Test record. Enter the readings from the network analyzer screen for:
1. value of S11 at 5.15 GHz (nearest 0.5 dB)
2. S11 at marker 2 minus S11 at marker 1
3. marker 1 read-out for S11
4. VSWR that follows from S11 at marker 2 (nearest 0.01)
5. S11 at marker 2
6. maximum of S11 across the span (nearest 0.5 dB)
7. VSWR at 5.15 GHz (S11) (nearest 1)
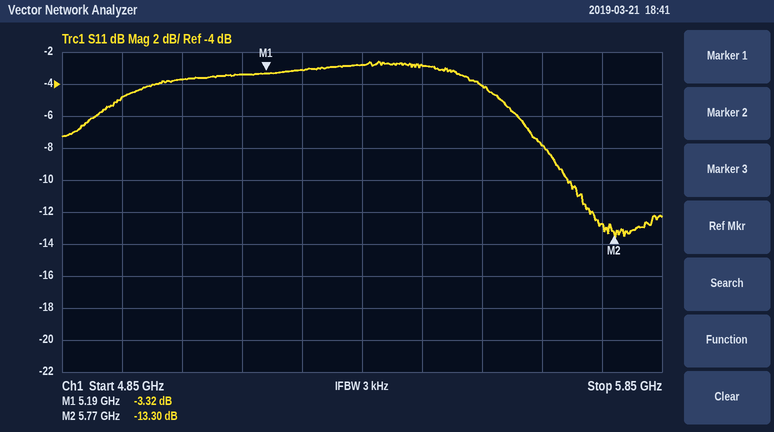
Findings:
-3.5 dB
-9.98 dB
-3.32 dB
1.55
-13.30 dB
-2.5 dB
5
